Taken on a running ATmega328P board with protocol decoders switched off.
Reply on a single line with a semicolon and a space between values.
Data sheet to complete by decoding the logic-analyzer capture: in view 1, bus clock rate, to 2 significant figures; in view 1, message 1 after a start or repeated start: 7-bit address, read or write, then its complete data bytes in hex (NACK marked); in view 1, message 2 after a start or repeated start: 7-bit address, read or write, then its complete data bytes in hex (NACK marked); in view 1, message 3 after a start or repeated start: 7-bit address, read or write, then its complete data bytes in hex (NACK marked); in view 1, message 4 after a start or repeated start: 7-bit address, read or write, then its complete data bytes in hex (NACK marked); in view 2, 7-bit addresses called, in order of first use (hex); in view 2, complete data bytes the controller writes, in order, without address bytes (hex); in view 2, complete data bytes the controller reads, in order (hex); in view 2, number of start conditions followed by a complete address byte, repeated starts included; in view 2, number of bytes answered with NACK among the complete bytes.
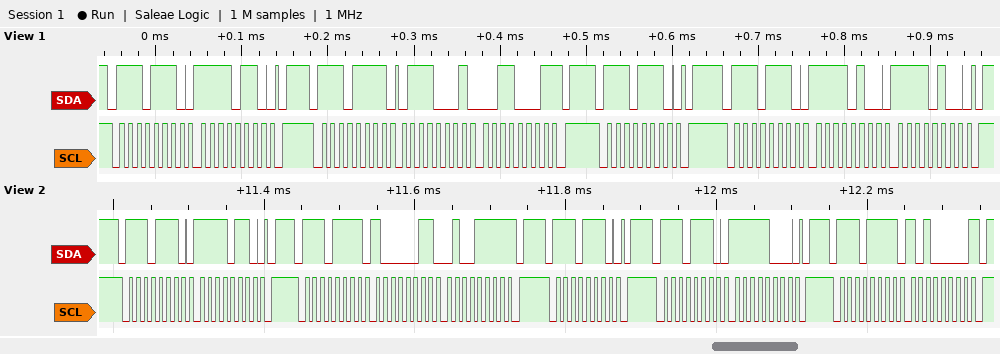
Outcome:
100 kHz; 0x77 write: F6; 0x77 read: 71 31 NACK; 0x77 write; 0x77 write: F4 F4; 0x77; F6 F8; 83 4F A0; 5; 2
